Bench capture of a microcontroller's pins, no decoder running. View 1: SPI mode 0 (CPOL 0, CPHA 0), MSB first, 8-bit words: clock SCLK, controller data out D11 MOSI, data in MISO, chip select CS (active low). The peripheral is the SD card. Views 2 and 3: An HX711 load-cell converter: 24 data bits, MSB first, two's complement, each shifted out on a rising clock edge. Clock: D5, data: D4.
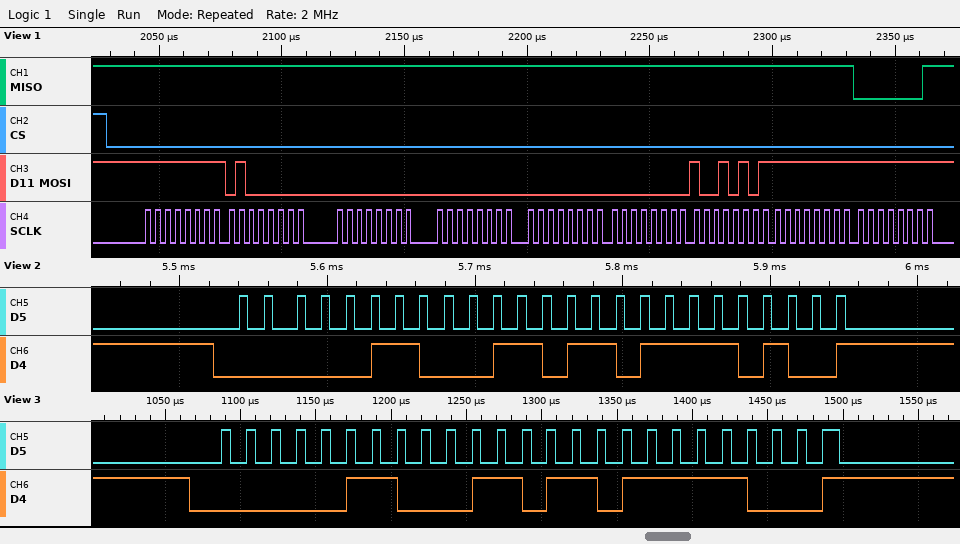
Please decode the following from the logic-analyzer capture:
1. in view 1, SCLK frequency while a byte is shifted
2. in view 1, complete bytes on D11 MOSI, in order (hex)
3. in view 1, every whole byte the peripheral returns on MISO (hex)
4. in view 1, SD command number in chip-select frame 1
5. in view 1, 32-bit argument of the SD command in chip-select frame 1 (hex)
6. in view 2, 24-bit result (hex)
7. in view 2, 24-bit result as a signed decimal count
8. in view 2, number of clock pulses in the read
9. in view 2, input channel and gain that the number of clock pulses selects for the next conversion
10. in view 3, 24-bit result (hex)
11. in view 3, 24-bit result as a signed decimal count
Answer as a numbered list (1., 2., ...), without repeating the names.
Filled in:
1. 250 kHz
2. 0xFF 0x40 0x00 0x00 0x00 0x00 0x95 0xFF 0xFF
3. 0xFF 0xFF 0xFF 0xFF 0xFF 0xFF 0xFF 0xFF 0x01
4. CMD0
5. 0x00000000
6. 0x0636F4
7. 407284
8. 25
9. channel A, gain 128
10. 0x0636F8
11. 407288
